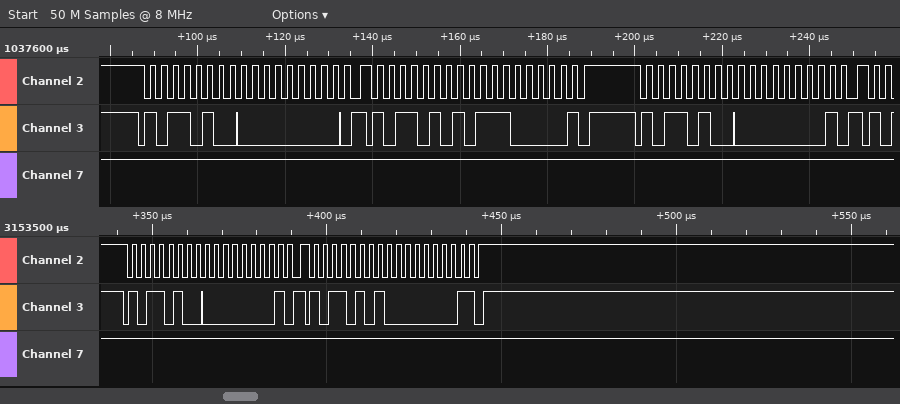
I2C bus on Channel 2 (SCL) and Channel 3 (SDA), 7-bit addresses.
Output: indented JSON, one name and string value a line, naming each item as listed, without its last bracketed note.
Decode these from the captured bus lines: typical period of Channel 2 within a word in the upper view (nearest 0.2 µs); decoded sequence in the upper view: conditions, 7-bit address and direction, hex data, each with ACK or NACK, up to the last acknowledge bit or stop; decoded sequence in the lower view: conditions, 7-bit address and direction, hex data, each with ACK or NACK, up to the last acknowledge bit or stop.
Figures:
{
  "typical period of Channel 2 within a word in the upper view": "2.6 µs",
  "decoded sequence in the upper view: conditions, 7-bit address and direction, hex data, each with ACK or NACK, up to the last acknowledge bit or stop": "start, address 5A write ACK, 00 ACK, repeated start, address 5A read ACK, E0 NACK, stop, start, address 5A write ACK, 01 ACK",
  "decoded sequence in the lower view: conditions, 7-bit address and direction, hex data, each with ACK or NACK, up to the last acknowledge bit or stop": "start, address 5A write ACK, 01 ACK, repeated start, address 5A read ACK, 01 NACK, stop"
}
